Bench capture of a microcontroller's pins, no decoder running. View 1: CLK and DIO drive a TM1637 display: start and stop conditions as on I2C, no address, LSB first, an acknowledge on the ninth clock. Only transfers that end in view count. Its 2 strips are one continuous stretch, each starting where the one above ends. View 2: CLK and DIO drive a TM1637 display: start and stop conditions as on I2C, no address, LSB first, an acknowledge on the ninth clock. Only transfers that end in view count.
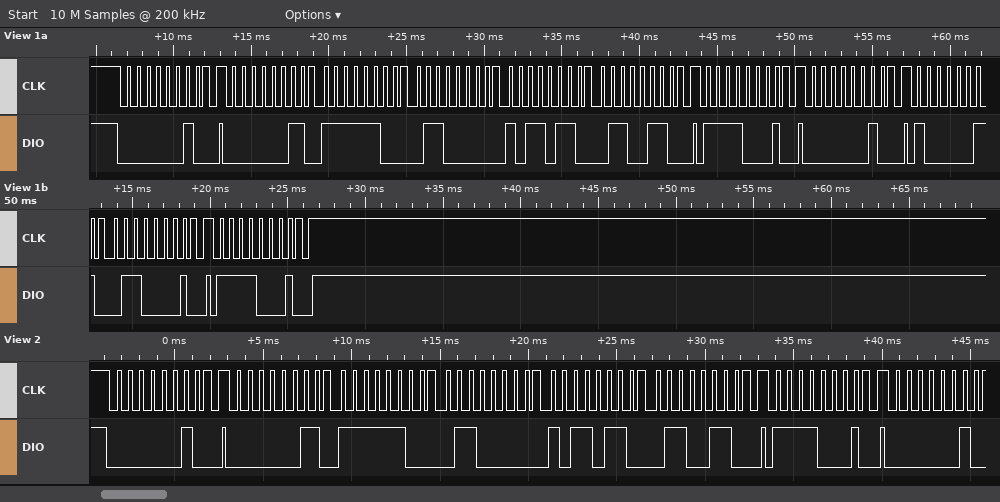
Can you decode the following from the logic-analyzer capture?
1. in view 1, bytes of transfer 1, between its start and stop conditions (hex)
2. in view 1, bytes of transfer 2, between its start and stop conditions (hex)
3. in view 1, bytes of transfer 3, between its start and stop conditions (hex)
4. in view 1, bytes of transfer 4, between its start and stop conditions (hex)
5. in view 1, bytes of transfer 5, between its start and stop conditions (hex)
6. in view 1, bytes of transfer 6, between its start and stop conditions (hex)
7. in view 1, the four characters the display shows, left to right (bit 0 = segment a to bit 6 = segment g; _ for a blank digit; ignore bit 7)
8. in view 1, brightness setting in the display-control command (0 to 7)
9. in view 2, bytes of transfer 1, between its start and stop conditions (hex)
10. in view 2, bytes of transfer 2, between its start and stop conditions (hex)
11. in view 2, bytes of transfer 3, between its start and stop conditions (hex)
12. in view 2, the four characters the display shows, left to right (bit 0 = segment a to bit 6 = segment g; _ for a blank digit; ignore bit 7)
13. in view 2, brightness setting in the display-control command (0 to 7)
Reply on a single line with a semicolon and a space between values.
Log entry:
40; C0 3F 06 6D 66; 8F; 40; C1 86; 8F; 0154; 7; 40; C0 3F 06 6D 66; 8F; 0154; 7
